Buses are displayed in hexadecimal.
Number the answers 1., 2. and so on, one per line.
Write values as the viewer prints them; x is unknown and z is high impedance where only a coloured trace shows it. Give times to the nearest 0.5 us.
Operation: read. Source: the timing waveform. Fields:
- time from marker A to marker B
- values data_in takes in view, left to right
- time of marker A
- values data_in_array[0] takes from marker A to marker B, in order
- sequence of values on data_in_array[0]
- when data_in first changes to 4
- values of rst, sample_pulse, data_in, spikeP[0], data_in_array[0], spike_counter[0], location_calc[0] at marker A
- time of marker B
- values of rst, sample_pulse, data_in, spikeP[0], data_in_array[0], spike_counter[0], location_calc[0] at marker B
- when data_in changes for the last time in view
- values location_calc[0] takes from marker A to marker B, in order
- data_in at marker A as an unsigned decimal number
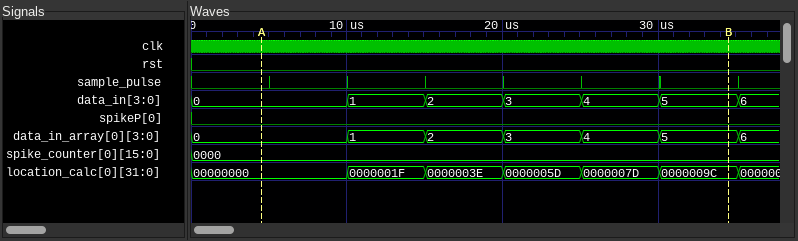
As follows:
1. 30 us
2. 0, 1, 2, 3, 4, 5, 6
3. 4.5 us
4. 0, 1, 2, 3, 4, 5
5. 0, 1, 2, 3, 4, 5, 6
6. 25 us
7. rst=0, sample_pulse=0, data_in=0, spikeP[0]=0, data_in_array[0]=0, spike_counter[0]=0000, location_calc[0]=00000000
8. 34.5 us
9. rst=0, sample_pulse=0, data_in=5, spikeP[0]=0, data_in_array[0]=5, spike_counter[0]=0000, location_calc[0]=0000009C
10. 35 us
11. 00000000, 0000001F, 0000003E, 0000005D, 0000007D, 0000009C
12. 0
